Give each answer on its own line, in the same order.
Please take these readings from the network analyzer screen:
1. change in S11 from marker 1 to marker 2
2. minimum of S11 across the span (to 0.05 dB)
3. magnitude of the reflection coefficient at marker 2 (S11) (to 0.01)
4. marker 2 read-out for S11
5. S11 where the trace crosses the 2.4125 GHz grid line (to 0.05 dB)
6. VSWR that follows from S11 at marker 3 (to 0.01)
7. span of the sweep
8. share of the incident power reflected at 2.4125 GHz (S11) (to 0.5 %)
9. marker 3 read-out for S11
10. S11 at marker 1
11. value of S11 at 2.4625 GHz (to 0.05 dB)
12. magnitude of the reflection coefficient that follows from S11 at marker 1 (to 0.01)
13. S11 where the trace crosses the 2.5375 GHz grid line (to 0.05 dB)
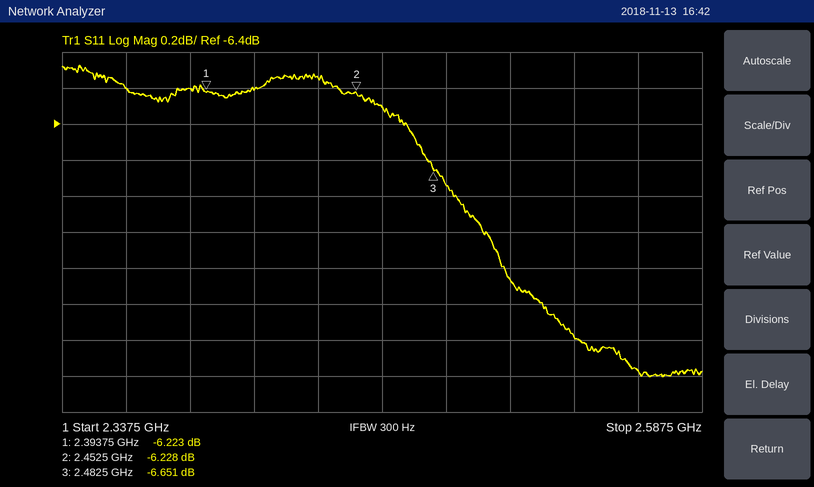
-0.005 dB
-7.80 dB
0.49
-6.228 dB
-6.20 dB
2.74
250 MHz
24.0 %
-6.651 dB
-6.223 dB
-6.30 dB
0.49
-7.60 dB
